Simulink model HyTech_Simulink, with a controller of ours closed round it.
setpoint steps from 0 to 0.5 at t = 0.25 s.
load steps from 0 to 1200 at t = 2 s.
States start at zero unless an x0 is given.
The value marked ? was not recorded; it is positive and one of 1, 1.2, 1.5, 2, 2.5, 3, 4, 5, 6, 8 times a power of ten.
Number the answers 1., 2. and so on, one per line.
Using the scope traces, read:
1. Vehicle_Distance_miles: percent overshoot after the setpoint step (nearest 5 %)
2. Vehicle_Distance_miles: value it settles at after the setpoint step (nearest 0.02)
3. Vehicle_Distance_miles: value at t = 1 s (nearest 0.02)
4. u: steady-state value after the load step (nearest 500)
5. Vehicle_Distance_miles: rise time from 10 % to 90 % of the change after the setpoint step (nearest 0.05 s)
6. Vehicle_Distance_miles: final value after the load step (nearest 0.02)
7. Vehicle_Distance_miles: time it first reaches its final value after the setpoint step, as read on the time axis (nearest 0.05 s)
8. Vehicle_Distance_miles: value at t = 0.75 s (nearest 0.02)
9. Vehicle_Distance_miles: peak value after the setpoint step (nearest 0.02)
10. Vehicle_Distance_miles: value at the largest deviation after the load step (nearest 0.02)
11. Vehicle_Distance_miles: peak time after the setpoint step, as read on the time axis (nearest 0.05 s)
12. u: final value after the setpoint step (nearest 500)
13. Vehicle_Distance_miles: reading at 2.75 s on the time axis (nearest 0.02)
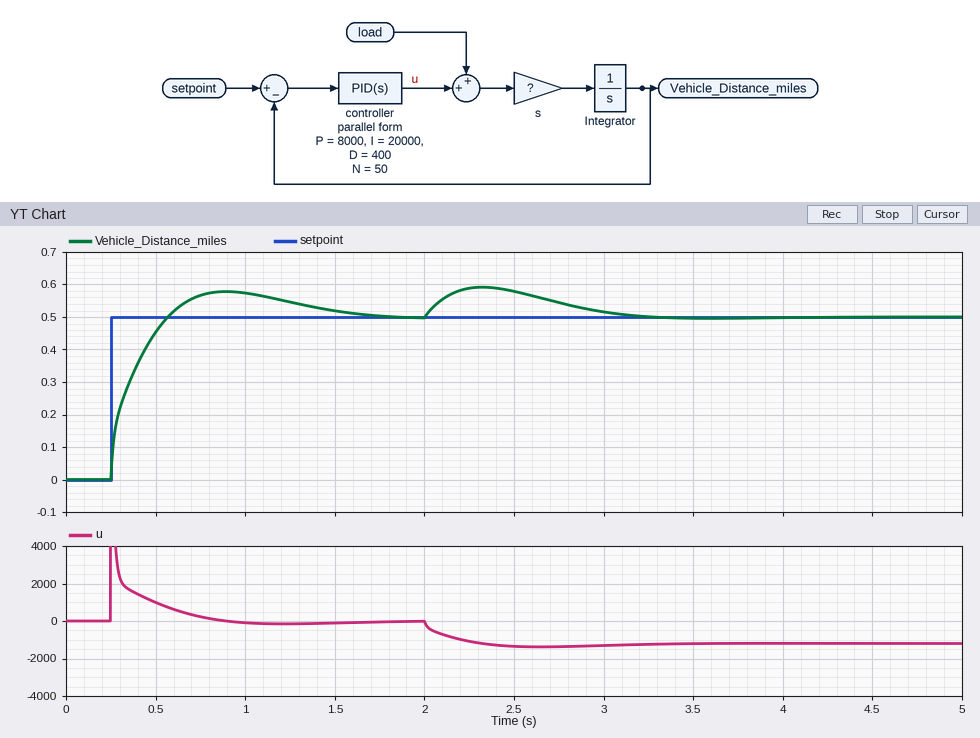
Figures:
1. 15 %
2. 0.50
3. 0.58
4. -1000
5. 0.25 s
6. 0.50
7. 0.55 s
8. 0.56
9. 0.58
10. 0.60
11. 0.90 s
12. 0
13. 0.54
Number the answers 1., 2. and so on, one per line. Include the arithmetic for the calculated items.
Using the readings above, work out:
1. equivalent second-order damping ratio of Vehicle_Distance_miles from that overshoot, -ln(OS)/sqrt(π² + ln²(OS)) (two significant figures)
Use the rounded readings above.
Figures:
1. ln(0.15) = -1.897; 1.897 / sqrt(9.870 + 3.599) = 0.52
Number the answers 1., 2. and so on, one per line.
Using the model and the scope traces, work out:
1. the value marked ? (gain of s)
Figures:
1. 0.0008
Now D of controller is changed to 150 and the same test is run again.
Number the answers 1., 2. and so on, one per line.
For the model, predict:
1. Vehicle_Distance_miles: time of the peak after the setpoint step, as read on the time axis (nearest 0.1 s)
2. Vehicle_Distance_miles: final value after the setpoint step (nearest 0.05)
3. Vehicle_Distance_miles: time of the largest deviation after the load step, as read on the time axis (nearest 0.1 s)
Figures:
1. 0.8 s
2. 0.50
3. 2.3 s
